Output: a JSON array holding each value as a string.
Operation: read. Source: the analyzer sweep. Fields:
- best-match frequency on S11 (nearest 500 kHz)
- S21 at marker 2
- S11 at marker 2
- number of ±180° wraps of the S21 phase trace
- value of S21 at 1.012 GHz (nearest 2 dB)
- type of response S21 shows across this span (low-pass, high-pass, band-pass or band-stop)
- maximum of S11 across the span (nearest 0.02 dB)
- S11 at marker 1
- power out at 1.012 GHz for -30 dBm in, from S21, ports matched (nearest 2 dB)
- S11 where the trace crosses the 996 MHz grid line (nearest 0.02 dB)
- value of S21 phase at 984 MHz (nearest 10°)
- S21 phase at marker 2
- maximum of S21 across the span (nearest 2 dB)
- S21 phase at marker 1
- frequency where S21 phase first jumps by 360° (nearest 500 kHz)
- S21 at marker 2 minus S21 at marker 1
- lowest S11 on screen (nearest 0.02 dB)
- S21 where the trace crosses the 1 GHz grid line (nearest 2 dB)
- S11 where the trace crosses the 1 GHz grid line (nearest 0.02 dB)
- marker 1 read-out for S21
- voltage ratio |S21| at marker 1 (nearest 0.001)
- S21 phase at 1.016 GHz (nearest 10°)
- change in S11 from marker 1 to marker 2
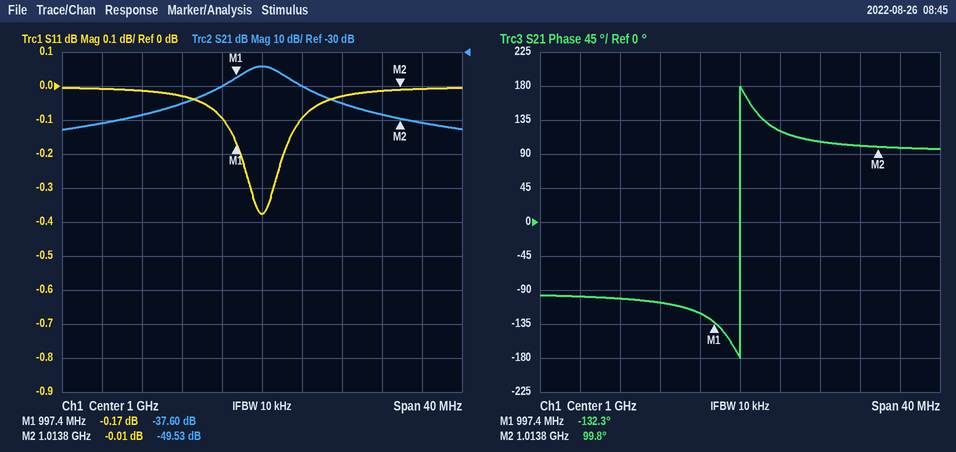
["1.0000 GHz", "-49.53 dB", "-0.01 dB", "1", "-48 dB", "band-pass", "0.00 dB", "-0.17 dB", "-78 dBm", "-0.10 dB", "-100°", "99.8°", "-34 dB", "-132.3°", "1.0000 GHz", "-11.93 dB", "-0.38 dB", "-34 dB", "-0.38 dB", "-37.60 dB", "0.013", "100°", "0.16 dB"]
